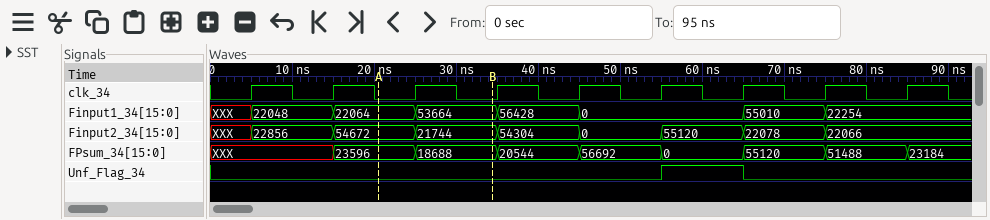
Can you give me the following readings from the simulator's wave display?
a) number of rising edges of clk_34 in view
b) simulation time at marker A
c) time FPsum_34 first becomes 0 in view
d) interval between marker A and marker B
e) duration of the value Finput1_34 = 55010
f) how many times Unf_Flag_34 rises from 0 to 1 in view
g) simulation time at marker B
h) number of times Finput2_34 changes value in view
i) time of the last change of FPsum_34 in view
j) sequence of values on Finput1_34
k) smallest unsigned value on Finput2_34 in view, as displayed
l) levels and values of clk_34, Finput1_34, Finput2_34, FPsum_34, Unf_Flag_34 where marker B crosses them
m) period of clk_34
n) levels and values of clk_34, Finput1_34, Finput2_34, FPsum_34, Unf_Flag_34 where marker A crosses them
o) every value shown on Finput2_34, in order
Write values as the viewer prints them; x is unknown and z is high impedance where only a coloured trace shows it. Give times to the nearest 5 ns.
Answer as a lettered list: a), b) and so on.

a) 9
b) 20 ns
c) 55 ns
d) 15 ns
e) 10 ns
f) 1
g) 35 ns
h) 8
i) 85 ns
j) XXX, 22048, 22064, 53664, 56428, 0, 55010, 22254
k) 0
l) clk_34=0, Finput1_34=53664, Finput2_34=21744, FPsum_34=18688, Unf_Flag_34=0
m) 10 ns
n) clk_34=0, Finput1_34=22064, Finput2_34=54672, FPsum_34=23596, Unf_Flag_34=0
o) XXX, 22856, 54672, 21744, 54304, 0, 55120, 22078, 22066
